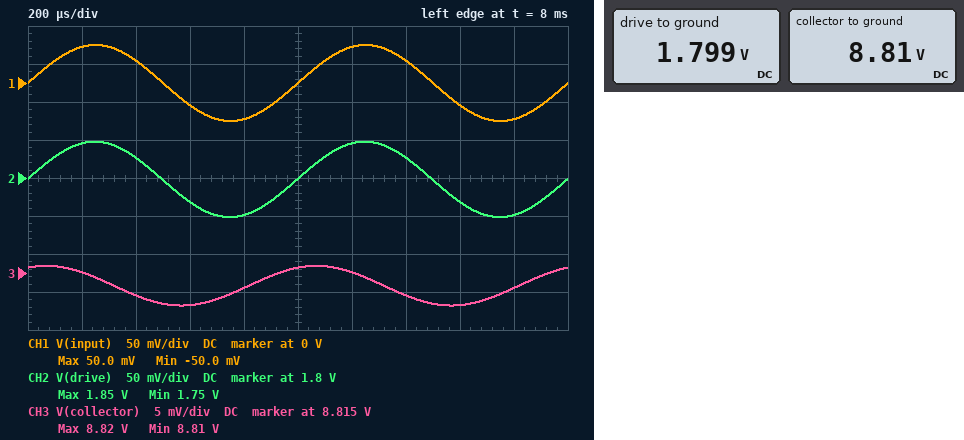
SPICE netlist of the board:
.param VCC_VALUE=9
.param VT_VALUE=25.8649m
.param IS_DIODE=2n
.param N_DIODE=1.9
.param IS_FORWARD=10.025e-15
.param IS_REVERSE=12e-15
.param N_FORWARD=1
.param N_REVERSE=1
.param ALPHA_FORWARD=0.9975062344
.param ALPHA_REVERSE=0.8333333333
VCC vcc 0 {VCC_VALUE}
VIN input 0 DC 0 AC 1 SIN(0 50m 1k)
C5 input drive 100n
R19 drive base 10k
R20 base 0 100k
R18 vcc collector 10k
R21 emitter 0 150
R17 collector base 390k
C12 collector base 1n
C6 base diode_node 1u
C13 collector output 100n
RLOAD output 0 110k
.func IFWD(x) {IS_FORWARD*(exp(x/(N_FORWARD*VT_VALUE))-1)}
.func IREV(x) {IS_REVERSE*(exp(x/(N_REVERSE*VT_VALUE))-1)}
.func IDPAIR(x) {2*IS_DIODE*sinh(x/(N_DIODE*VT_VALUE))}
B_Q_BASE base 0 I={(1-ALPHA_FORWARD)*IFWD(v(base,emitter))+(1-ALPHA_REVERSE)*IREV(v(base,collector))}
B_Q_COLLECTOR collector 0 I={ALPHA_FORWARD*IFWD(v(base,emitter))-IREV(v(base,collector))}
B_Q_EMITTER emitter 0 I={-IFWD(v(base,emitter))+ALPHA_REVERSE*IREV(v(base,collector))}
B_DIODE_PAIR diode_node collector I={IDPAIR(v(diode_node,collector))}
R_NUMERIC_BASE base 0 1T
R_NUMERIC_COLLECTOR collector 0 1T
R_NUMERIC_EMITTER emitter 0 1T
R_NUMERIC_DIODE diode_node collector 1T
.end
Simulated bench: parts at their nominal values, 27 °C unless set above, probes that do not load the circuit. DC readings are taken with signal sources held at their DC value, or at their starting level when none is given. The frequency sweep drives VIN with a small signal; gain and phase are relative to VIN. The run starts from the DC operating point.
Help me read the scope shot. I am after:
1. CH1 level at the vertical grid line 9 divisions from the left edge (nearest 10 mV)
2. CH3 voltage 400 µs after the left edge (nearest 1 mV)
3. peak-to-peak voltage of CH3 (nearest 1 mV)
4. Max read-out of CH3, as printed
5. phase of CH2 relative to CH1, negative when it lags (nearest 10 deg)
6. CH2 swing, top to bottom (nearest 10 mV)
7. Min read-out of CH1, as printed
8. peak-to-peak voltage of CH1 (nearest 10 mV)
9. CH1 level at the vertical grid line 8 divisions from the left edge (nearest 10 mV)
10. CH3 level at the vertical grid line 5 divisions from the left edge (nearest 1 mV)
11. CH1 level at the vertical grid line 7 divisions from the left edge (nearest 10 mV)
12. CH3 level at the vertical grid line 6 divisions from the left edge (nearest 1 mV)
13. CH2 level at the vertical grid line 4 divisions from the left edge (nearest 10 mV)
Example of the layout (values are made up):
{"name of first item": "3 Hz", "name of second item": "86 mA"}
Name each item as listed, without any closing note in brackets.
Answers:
{"CH1 level at the vertical grid line 9 divisions from the left edge": "-50 mV", "CH3 voltage 400 µs after the left edge": "8.812 V", "peak-to-peak voltage of CH3": "5 mV", "Max read-out of CH3, as printed": "8.82 V", "phase of CH2 relative to CH1, negative when it lags": "0 deg", "CH2 swing, top to bottom": "100 mV", "Min read-out of CH1, as printed": "-50.0 mV", "peak-to-peak voltage of CH1": "100 mV", "CH1 level at the vertical grid line 8 divisions from the left edge": "-30 mV", "CH3 level at the vertical grid line 5 divisions from the left edge": "8.816 V", "CH1 level at the vertical grid line 7 divisions from the left edge": "30 mV", "CH3 level at the vertical grid line 6 divisions from the left edge": "8.815 V", "CH2 level at the vertical grid line 4 divisions from the left edge": "1.75 V"}
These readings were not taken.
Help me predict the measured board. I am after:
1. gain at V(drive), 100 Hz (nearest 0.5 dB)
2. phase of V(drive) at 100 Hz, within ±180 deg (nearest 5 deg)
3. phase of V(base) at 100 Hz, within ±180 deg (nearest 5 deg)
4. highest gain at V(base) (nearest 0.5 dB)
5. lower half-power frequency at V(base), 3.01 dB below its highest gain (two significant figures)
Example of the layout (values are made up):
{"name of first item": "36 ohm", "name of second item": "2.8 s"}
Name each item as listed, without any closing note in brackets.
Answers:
{"gain at V(drive), 100 Hz": "0 dB", "phase of V(drive) at 100 Hz, within ±180 deg": "10 deg", "phase of V(base) at 100 Hz, within ±180 deg": "10 deg", "highest gain at V(base)": "-1.0 dB", "lower half-power frequency at V(base), 3.01 dB below its highest gain": "18 Hz"}
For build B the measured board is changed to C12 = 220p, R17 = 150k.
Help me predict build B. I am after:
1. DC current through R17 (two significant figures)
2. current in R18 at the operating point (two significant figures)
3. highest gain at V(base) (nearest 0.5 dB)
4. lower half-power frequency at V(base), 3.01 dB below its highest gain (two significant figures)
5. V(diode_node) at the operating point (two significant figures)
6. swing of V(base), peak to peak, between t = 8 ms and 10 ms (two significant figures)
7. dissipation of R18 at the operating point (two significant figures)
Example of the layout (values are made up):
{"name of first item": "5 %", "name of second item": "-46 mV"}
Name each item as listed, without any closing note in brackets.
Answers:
{"DC current through R17": "35 µA", "current in R18 at the operating point": "36 µA", "highest gain at V(base)": "-1.5 dB", "lower half-power frequency at V(base), 3.01 dB below its highest gain": "22 Hz", "V(diode_node) at the operating point": "8.6 V", "swing of V(base), peak to peak, between t = 8 ms and 10 ms": "86 mV", "dissipation of R18 at the operating point": "13 µW"}
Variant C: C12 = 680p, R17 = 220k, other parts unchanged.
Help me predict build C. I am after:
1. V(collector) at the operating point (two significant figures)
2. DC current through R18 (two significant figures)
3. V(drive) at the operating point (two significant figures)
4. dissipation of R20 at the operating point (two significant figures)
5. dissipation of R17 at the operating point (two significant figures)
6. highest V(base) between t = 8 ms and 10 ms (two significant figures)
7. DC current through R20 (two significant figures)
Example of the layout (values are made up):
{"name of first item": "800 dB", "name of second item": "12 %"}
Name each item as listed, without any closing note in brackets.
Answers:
{"V(collector) at the operating point": "8.7 V", "DC current through R18": "28 µA", "V(drive) at the operating point": "2.7 V", "dissipation of R20 at the operating point": "74 µW", "dissipation of R17 at the operating point": "160 µW", "highest V(base) between t = 8 ms and 10 ms": "2.8 V", "DC current through R20": "27 µA"}
